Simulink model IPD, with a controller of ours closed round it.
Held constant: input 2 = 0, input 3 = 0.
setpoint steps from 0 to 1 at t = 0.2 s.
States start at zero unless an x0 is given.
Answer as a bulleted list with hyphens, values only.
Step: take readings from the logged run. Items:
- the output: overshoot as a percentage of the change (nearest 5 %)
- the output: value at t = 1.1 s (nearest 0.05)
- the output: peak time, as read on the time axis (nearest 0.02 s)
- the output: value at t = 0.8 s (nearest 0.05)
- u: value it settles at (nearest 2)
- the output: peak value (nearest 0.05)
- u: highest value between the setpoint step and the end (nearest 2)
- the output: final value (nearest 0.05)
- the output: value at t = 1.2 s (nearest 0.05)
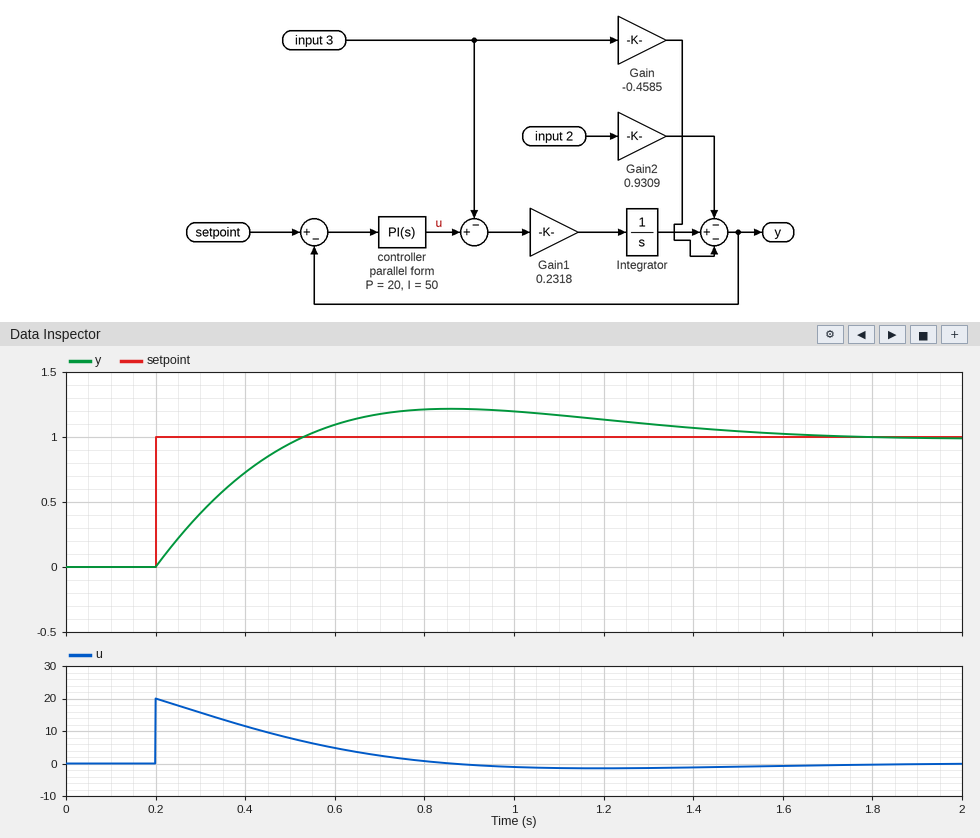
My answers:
- 20 %
- 1.15
- 0.86 s
- 1.20
- 0
- 1.20
- 20
- 1.00
- 1.15
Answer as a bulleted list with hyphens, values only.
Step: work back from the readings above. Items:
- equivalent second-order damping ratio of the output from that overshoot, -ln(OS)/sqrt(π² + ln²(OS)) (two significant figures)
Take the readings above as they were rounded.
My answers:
- 0.46
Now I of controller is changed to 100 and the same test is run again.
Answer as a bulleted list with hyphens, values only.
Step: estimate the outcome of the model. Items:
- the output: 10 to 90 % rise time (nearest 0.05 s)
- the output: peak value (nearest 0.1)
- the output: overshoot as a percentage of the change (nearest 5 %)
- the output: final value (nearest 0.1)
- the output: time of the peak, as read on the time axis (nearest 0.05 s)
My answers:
- 0.20 s
- 1.3
- 30 %
- 1.0
- 0.70 s
